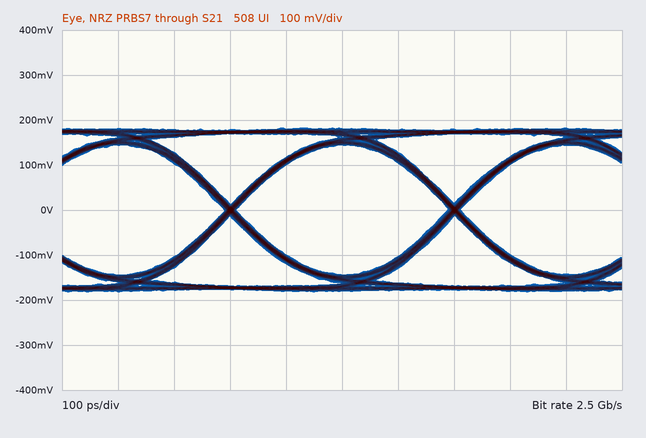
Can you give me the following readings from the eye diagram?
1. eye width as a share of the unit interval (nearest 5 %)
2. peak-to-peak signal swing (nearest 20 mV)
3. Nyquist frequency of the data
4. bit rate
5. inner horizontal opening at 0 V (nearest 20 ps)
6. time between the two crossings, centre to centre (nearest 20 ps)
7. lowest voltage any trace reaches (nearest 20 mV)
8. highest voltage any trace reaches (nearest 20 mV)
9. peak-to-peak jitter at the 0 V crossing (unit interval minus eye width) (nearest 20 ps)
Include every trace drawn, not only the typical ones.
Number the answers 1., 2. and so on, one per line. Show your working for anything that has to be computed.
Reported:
1. 380 ps / 400 ps ≈ 95 %
2. 360 mV
3. 1.25 GHz
4. 2.5 Gb/s
5. 380 ps
6. 400 ps
7. -180 mV
8. 180 mV
9. 20 ps
